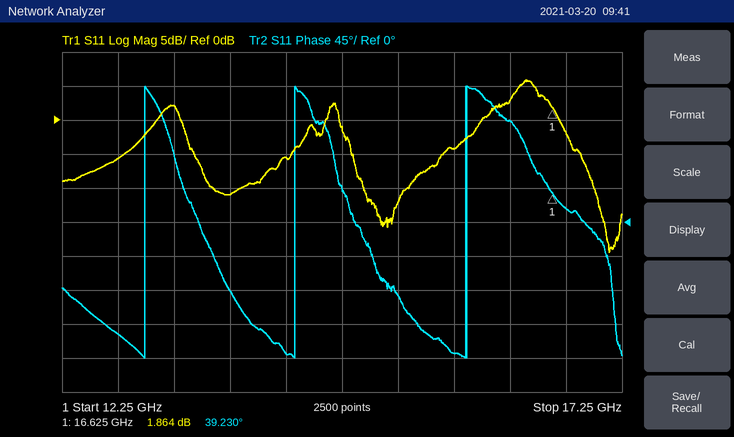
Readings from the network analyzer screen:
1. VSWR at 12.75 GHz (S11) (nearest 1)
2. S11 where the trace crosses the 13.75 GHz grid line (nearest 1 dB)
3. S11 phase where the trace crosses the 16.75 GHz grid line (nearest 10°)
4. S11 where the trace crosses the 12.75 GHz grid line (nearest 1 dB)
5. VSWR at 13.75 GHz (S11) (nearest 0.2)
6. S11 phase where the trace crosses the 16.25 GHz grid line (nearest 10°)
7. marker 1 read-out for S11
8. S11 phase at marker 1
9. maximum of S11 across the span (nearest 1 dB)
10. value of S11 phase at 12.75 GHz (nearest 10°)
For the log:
3
-11 dB
20°
-6 dB
1.8
130°
1.864 dB
39.230°
6 dB
-150°
